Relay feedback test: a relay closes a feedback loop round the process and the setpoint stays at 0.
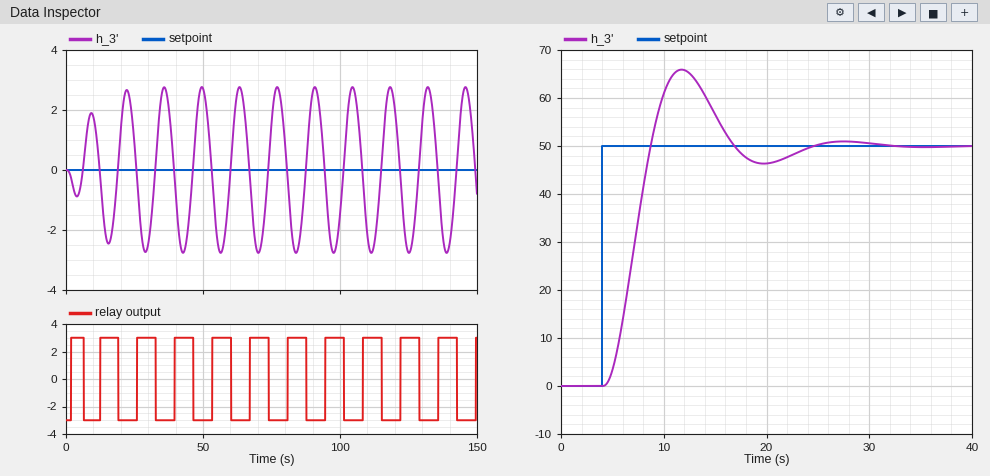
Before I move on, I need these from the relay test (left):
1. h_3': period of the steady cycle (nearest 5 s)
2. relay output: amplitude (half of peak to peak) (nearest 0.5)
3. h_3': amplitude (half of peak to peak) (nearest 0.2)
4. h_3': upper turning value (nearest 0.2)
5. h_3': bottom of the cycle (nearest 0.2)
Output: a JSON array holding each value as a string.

["15 s", "3.0", "2.8", "2.8", "-2.8"]
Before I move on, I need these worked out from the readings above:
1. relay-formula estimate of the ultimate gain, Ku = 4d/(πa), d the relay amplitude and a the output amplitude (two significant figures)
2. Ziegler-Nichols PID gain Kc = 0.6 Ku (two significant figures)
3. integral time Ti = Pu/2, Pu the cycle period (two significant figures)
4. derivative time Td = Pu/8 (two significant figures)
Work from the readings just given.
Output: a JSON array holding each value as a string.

["1.4", "0.84", "7.5 s", "1.9 s"]
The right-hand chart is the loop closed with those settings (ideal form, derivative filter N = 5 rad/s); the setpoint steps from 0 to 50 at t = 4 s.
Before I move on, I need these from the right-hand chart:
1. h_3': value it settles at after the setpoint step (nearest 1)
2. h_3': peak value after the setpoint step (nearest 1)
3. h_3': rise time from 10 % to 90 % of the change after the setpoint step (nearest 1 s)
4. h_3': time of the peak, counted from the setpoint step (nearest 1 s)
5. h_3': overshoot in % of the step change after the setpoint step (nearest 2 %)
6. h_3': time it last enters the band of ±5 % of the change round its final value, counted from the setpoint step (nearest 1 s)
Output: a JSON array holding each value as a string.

["50", "66", "3 s", "8 s", "32 %", "18 s"]
